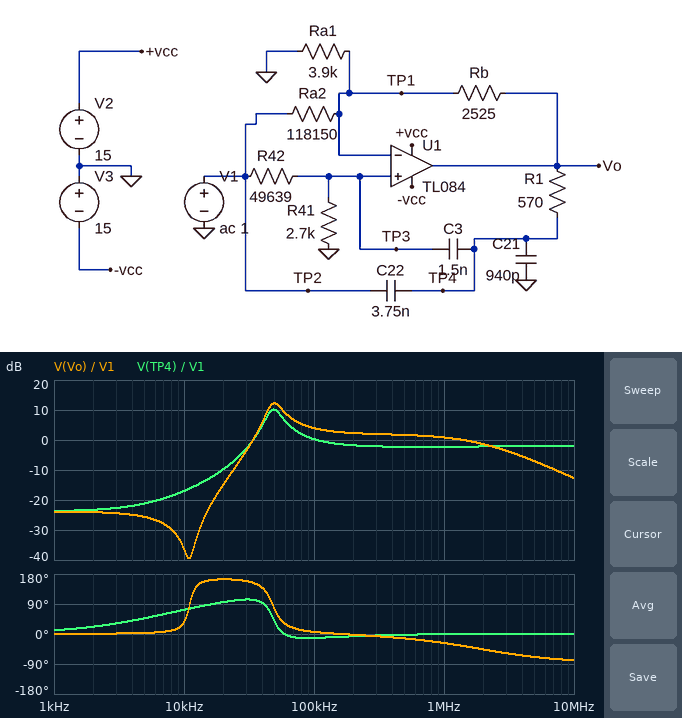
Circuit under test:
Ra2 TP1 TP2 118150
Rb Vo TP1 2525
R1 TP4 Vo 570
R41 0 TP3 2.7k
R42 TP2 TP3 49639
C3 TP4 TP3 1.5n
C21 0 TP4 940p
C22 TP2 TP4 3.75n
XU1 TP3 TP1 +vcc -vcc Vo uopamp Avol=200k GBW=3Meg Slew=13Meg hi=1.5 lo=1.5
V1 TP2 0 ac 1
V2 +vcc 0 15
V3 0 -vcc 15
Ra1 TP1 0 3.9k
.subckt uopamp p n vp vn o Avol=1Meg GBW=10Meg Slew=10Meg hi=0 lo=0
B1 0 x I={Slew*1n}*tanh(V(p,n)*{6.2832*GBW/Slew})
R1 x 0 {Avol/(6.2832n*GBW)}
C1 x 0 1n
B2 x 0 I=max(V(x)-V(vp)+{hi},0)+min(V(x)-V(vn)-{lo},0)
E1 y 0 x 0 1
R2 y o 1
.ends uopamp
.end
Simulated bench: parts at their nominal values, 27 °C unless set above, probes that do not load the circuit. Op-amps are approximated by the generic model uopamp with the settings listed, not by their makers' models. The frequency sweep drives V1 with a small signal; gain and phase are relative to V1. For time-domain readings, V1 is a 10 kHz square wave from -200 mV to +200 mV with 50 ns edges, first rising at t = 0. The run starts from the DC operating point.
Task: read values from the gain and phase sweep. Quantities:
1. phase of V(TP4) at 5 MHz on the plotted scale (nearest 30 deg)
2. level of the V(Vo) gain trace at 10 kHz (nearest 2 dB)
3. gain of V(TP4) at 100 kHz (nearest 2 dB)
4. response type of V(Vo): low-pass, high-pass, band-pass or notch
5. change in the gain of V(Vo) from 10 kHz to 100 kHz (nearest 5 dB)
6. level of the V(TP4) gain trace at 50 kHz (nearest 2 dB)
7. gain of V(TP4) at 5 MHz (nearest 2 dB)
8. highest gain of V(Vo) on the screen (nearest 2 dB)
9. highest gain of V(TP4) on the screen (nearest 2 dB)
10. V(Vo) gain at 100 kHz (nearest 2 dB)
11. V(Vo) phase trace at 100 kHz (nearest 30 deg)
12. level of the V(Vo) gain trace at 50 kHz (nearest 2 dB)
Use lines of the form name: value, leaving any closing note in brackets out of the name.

phase of V(TP4) at 5 MHz on the plotted scale: 0 deg
level of the V(Vo) gain trace at 10 kHz: -36 dB
gain of V(TP4) at 100 kHz: 0 dB
response type of V(Vo): low-pass, high-pass, band-pass or notch: band-pass
change in the gain of V(Vo) from 10 kHz to 100 kHz: 40 dB
level of the V(TP4) gain trace at 50 kHz: 10 dB
gain of V(TP4) at 5 MHz: -2 dB
highest gain of V(Vo) on the screen: 12 dB
highest gain of V(TP4) on the screen: 10 dB
V(Vo) gain at 100 kHz: 4 dB
V(Vo) phase trace at 100 kHz: 0 deg
level of the V(Vo) gain trace at 50 kHz: 12 dB
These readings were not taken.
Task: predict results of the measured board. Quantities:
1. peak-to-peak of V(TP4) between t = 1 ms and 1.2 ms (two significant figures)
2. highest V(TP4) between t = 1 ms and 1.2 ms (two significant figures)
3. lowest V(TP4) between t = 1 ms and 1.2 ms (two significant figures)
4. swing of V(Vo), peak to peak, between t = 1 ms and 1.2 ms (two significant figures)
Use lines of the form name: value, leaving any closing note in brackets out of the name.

peak-to-peak of V(TP4) between t = 1 ms and 1.2 ms: 710 mV
highest V(TP4) between t = 1 ms and 1.2 ms: 360 mV
lowest V(TP4) between t = 1 ms and 1.2 ms: -360 mV
swing of V(Vo), peak to peak, between t = 1 ms and 1.2 ms: 1.0 V
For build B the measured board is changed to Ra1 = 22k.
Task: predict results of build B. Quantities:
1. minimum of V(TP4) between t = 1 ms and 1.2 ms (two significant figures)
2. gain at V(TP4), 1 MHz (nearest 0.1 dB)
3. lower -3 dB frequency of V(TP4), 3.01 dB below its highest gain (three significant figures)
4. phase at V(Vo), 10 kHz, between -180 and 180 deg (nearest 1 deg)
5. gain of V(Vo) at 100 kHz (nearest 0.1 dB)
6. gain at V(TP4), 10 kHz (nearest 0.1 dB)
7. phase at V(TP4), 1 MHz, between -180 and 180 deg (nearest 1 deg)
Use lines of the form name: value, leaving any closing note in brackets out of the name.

minimum of V(TP4) between t = 1 ms and 1.2 ms: -310 mV
gain at V(TP4), 1 MHz: -2.1 dB
lower -3 dB frequency of V(TP4), 3.01 dB below its highest gain: 37.5 kHz
phase at V(Vo), 10 kHz, between -180 and 180 deg: 56 deg
gain of V(Vo) at 100 kHz: -0.3 dB
gain at V(TP4), 10 kHz: -17.4 dB
phase at V(TP4), 1 MHz, between -180 and 180 deg: 1 deg
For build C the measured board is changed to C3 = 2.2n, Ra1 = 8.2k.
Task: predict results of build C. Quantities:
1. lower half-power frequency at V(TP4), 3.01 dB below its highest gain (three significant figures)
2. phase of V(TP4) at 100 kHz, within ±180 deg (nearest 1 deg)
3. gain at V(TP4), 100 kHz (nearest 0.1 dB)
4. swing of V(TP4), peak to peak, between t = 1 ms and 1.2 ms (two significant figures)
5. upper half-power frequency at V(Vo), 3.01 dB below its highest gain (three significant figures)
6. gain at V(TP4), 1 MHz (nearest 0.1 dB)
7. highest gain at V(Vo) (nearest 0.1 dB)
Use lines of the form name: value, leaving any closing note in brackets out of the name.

lower half-power frequency at V(TP4), 3.01 dB below its highest gain: 33.6 kHz
phase of V(TP4) at 100 kHz, within ±180 deg: -1 deg
gain at V(TP4), 100 kHz: -0.7 dB
swing of V(TP4), peak to peak, between t = 1 ms and 1.2 ms: 600 mV
upper half-power frequency at V(Vo), 3.01 dB below its highest gain: 70.2 kHz
gain at V(TP4), 1 MHz: -2.2 dB
highest gain at V(Vo): 5.6 dB
